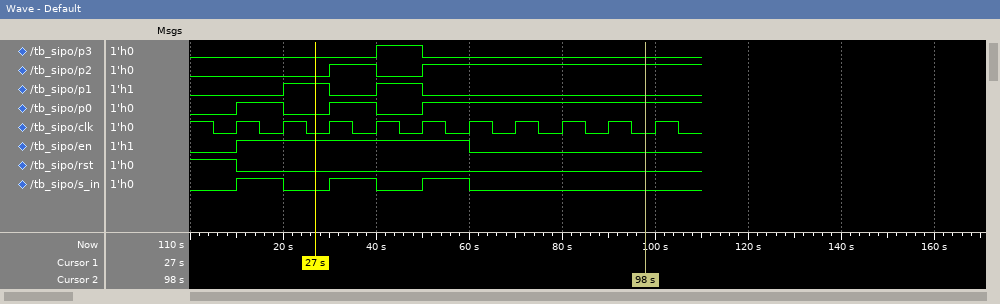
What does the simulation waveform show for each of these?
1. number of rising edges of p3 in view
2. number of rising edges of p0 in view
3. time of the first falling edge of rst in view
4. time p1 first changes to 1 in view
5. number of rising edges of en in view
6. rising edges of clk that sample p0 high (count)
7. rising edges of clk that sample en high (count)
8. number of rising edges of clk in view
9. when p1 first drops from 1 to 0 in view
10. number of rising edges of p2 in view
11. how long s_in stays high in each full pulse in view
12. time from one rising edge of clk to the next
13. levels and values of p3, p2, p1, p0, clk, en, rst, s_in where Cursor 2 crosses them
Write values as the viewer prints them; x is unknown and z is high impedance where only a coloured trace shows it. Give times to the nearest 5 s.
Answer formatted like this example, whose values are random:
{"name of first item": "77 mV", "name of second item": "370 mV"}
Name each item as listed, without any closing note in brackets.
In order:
{"number of rising edges of p3 in view": "1", "number of rising edges of p0 in view": "3", "time of the first falling edge of rst in view": "10 s", "time p1 first changes to 1 in view": "20 s", "number of rising edges of en in view": "1", "rising edges of clk that sample p0 high": "7", "rising edges of clk that sample en high": "5", "number of rising edges of clk in view": "10", "when p1 first drops from 1 to 0 in view": "30 s", "number of rising edges of p2 in view": "2", "how long s_in stays high in each full pulse in view": "10 s, 10 s, 10 s", "time from one rising edge of clk to the next": "10 s", "levels and values of p3, p2, p1, p0, clk, en, rst, s_in where Cursor 2 crosses them": "p3=0, p2=1, p1=0, p0=1, clk=0, en=0, rst=0, s_in=0"}
